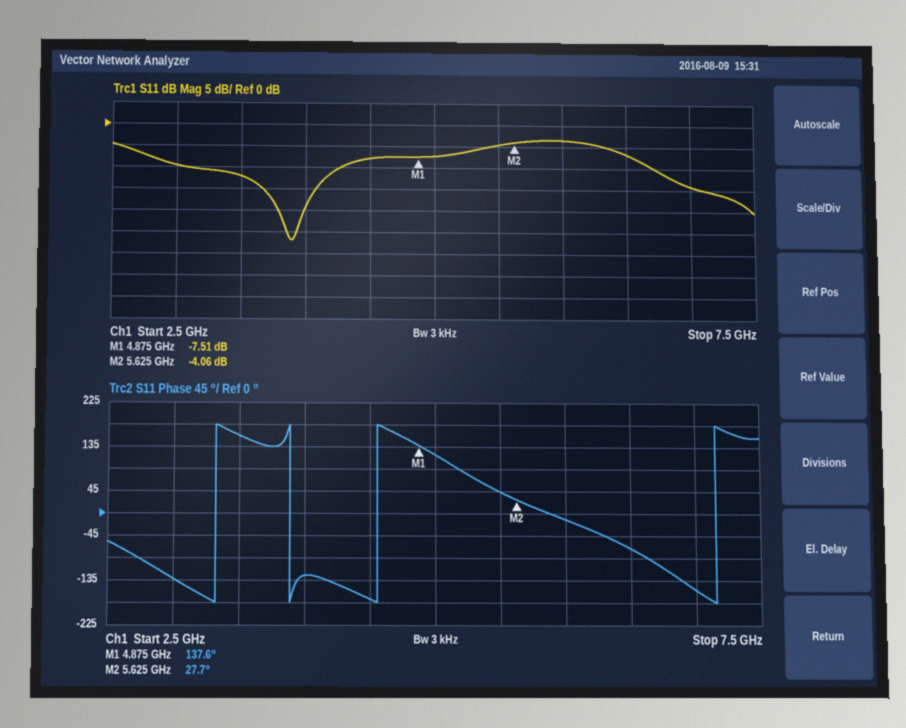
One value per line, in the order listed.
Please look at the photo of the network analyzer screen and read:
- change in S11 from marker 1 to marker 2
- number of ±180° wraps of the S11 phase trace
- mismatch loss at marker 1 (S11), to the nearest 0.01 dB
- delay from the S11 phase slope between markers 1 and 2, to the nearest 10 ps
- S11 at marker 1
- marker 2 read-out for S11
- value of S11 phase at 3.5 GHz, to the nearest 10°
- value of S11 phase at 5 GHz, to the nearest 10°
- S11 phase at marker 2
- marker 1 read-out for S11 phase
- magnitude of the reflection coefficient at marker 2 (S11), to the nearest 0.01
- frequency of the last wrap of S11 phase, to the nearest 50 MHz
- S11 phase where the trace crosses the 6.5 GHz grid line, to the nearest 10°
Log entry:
3.45 dB
4
0.85 dB
410 ps
-7.51 dB
-4.06 dB
160°
120°
27.7°
137.6°
0.63
7.15 GHz
-70°
